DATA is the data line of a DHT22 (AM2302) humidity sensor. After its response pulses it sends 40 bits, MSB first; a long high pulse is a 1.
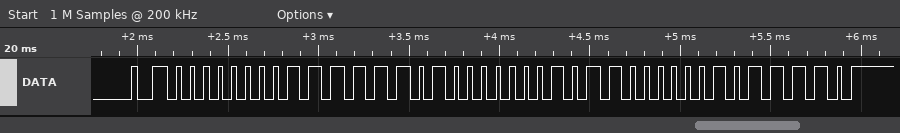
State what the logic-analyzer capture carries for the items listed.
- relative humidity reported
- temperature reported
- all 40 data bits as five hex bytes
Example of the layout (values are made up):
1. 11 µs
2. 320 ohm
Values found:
1. 25.3 %
2. 35.2 °C
3. 00 FD 01 60 5E
